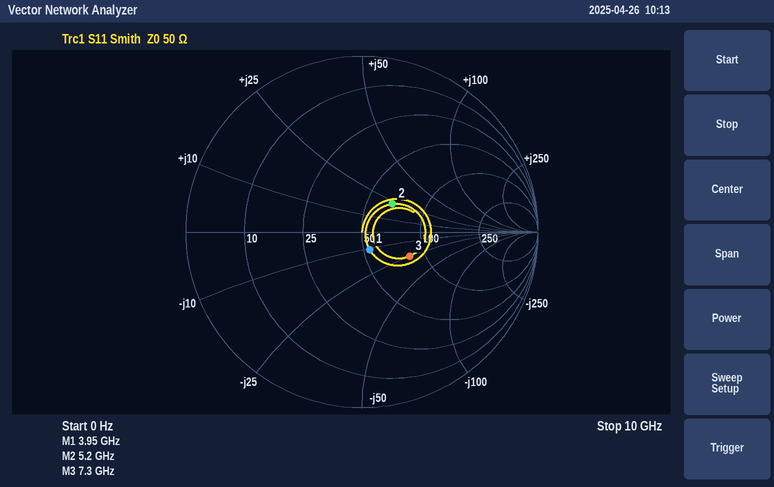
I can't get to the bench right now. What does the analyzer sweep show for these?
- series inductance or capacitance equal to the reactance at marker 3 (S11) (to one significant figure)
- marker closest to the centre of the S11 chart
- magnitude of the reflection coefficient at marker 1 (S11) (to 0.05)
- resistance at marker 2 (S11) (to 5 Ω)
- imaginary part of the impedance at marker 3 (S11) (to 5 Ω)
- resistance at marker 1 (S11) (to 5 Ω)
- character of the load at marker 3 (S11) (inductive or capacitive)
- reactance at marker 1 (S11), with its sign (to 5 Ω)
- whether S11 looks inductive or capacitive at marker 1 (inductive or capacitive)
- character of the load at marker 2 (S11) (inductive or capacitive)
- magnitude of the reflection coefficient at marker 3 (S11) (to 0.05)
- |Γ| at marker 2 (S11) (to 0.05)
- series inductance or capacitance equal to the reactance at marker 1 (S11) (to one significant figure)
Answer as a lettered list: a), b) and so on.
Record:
a) 900 fF
b) marker 1
c) 0.10
d) 65 Ω
e) -25 Ω
f) 55 Ω
g) capacitive
h) -10 Ω
i) capacitive
j) inductive
k) 0.30
l) 0.25
m) 4 pF
